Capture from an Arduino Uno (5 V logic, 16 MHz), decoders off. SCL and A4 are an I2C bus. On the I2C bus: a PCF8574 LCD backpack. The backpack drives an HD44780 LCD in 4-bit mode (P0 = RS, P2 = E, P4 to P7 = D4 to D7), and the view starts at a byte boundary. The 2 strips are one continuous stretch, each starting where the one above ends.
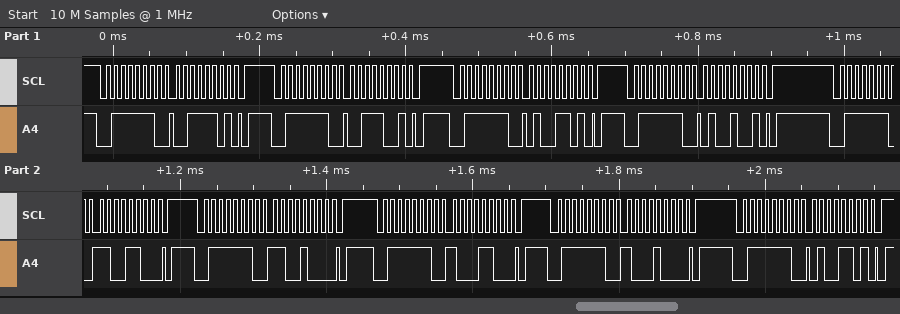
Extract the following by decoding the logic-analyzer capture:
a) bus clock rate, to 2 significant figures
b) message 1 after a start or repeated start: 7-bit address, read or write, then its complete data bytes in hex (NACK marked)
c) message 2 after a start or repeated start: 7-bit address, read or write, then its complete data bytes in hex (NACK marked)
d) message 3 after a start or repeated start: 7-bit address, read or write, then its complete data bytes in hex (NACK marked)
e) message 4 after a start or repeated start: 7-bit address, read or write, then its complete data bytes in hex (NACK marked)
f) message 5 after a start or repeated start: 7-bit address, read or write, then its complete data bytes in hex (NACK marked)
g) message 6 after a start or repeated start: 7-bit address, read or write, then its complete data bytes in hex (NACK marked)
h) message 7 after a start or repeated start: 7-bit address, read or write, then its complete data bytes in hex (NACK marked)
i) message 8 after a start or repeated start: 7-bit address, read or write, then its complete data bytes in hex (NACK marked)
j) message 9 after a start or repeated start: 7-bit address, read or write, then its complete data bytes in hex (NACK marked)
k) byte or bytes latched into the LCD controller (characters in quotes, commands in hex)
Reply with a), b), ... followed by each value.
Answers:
a) 100 kHz
b) 0x3F write: 3D
c) 0x3F write: 39
d) 0x3F write: 4D
e) 0x3F write: 49
f) 0x3F write: CC
g) 0x3F write: C8
h) 0x3F write: 8C
i) 0x3F write: 88
j) 0x3F write: 4D
k) '4' 0xC8
